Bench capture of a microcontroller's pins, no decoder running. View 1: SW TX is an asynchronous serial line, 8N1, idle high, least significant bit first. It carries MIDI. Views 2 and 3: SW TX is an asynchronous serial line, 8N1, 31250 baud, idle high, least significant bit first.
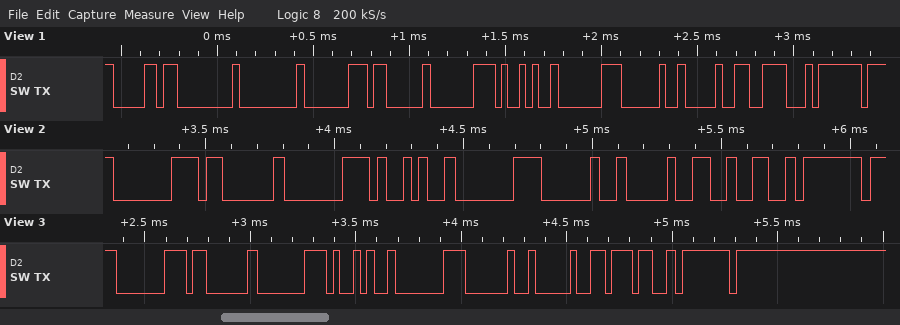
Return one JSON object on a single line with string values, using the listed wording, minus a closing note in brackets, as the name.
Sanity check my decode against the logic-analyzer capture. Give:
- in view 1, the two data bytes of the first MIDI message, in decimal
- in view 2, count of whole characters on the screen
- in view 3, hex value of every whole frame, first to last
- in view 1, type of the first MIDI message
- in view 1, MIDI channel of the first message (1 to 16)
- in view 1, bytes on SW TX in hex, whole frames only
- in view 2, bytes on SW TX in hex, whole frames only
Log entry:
{"in view 1, the two data bytes of the first MIDI message, in decimal": "0, 0", "in view 2, count of whole characters on the screen": "9", "in view 3, hex value of every whole frame, first to last": "0xC0 0x03 0xC0 0x29 0xC0 0x20 0x90 0x37 0x7F", "in view 1, type of the first MIDI message": "Control Change", "in view 1, MIDI channel of the first message": "1", "in view 1, bytes on SW TX in hex, whole frames only": "B0 00 00 C0 03 C0 29 C0 20 90 1E 7F", "in view 2, bytes on SW TX in hex, whole frames only": "0xC0 0x03 0xC0 0x29 0xC0 0x20 0x90 0x32 0x7F"}
